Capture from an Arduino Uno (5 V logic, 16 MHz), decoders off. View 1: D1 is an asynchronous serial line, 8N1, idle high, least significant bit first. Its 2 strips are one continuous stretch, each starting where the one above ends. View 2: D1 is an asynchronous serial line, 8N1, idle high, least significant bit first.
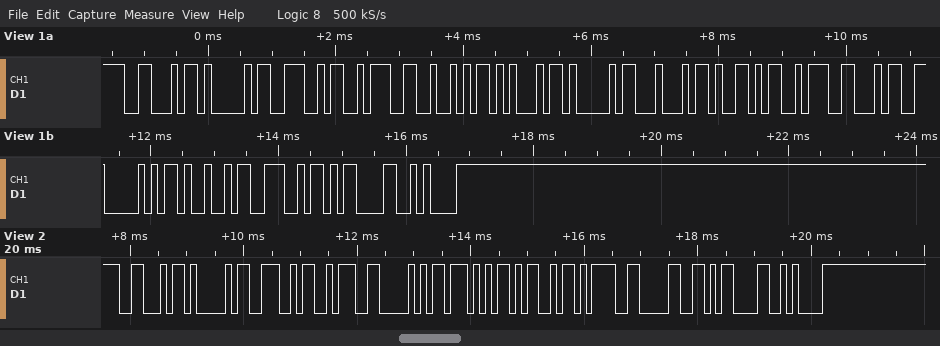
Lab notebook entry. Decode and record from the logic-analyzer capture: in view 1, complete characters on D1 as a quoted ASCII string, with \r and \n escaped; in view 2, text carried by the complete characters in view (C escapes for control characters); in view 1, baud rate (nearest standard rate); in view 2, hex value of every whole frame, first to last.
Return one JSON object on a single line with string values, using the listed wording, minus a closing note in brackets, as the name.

{"in view 1, complete characters on D1 as a quoted ASCII string, with \\r and \\n escaped": "\"FAN:READY:4PIN\\r\\n\"", "in view 2, text carried by the complete characters in view": "\"FAN:PWM=0\\r\\n\"", "in view 1, baud rate": "9600 baud", "in view 2, hex value of every whole frame, first to last": "46 41 4E 3A 50 57 4D 3D 30 0D 0A"}
